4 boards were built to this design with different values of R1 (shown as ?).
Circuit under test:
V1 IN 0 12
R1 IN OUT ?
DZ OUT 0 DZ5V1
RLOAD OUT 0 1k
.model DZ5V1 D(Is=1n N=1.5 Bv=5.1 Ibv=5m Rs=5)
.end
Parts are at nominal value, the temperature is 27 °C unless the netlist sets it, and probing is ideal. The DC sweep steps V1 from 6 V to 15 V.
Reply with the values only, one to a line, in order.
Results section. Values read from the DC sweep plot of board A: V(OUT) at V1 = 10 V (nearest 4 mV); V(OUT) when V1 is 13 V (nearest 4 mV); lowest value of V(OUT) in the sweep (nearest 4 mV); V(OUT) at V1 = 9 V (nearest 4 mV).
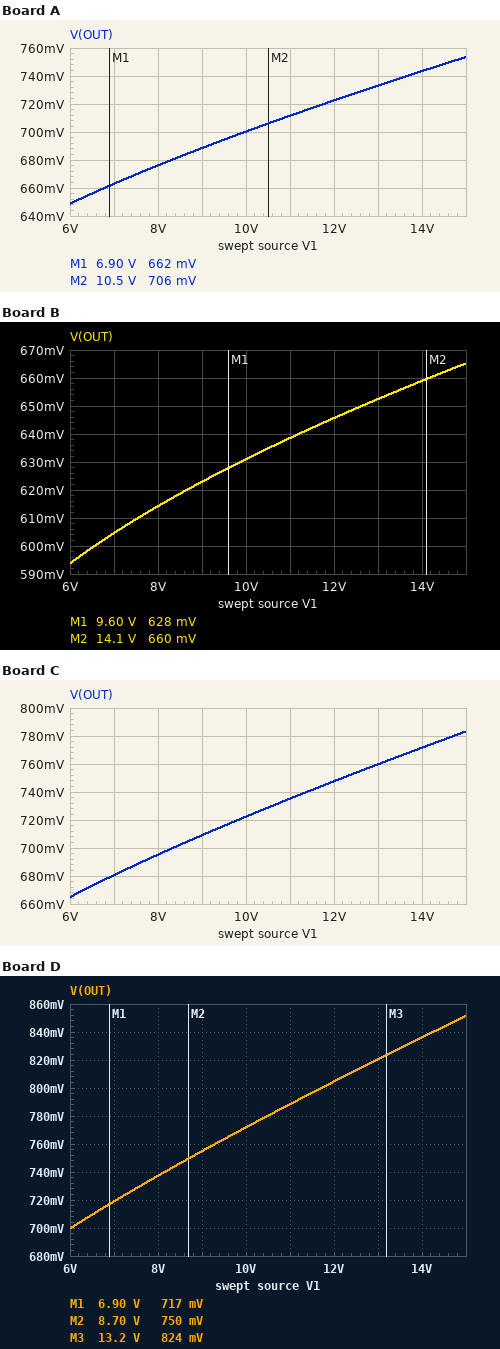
700 mV
732 mV
648 mV
688 mV
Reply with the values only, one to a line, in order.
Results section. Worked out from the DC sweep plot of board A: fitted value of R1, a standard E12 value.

680 Ω
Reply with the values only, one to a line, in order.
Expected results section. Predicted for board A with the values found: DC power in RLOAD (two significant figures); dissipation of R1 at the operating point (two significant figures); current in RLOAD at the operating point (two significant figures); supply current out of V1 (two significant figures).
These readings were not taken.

520 µW
190 mW
720 µA
17 mA
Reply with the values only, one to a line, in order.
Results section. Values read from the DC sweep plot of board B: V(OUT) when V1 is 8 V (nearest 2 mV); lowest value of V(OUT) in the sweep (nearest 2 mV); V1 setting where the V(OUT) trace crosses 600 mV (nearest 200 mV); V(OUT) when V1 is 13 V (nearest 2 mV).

614 mV
594 mV
6.6 V
652 mV
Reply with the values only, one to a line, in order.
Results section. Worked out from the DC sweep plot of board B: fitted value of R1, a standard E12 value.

1.5 kΩ
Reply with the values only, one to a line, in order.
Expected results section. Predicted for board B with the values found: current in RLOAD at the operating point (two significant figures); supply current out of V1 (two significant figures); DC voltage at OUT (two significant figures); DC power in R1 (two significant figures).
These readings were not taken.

650 µA
7.6 mA
650 mV
86 mW
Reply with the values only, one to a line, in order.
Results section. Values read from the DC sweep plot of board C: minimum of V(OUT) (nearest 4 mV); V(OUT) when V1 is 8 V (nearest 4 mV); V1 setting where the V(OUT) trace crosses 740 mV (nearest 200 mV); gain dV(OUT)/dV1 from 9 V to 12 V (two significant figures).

664 mV
696 mV
11.4 V
0.013 V/V
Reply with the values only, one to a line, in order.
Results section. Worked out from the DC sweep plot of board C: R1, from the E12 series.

560 Ω
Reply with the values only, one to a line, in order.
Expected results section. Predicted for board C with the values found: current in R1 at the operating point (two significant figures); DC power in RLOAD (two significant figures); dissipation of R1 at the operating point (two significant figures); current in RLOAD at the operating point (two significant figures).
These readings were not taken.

20 mA
560 µW
230 mW
750 µA
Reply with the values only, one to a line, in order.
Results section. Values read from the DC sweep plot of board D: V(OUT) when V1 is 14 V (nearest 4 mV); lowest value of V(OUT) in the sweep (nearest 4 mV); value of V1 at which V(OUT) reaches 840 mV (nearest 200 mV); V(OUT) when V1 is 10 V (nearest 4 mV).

836 mV
700 mV
14.2 V
772 mV
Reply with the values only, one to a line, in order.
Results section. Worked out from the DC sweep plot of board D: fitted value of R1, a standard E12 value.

390 Ω
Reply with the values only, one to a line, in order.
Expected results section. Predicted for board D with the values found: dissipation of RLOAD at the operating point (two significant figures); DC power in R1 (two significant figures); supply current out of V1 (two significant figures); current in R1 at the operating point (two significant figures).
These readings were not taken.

650 µW
320 mW
29 mA
29 mA
